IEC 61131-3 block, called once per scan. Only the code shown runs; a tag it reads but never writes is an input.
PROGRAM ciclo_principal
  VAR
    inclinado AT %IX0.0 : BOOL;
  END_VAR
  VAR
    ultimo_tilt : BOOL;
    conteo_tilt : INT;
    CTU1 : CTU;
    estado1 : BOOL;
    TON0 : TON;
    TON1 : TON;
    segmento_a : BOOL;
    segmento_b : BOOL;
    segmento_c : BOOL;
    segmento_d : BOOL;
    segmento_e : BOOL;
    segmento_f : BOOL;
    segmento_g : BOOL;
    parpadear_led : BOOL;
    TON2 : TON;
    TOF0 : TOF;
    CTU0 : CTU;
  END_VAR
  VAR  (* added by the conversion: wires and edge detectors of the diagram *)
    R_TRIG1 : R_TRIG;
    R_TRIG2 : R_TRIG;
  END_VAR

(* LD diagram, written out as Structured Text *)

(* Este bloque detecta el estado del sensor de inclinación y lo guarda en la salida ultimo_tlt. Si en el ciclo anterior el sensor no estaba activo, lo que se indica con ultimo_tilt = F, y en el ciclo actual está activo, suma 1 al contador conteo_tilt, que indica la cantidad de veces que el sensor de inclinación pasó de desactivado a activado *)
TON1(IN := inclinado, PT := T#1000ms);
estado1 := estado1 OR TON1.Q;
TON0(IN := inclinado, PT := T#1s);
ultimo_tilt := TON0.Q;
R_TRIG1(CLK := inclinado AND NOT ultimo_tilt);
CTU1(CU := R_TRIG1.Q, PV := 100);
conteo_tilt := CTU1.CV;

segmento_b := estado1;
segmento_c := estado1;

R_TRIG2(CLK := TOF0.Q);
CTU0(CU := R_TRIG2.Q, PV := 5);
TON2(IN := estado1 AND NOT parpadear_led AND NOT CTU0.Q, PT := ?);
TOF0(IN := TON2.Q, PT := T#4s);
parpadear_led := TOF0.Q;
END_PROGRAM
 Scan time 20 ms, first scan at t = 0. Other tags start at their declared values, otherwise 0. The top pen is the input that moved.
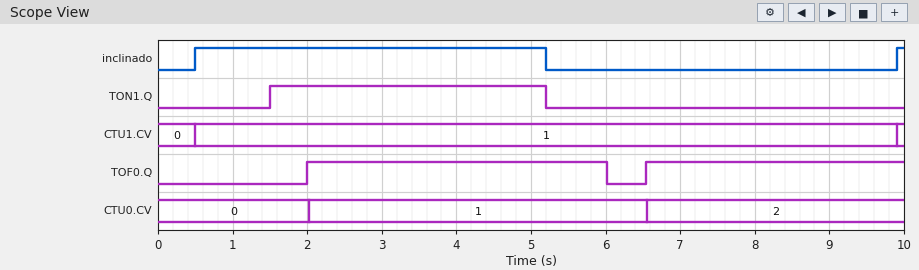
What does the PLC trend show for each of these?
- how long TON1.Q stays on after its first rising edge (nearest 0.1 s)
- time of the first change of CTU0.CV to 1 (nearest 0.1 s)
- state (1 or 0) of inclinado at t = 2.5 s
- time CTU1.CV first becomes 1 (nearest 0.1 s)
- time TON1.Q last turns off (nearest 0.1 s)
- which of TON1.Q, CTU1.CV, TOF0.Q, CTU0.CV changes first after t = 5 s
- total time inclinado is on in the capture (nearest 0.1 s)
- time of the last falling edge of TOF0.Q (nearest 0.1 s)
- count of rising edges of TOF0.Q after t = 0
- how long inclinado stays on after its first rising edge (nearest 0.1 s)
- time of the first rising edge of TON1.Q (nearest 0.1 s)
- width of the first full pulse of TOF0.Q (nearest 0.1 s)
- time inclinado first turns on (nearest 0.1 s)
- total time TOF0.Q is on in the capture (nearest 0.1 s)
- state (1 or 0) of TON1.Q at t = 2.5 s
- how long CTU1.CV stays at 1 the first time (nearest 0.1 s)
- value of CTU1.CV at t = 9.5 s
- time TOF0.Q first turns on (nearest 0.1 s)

3.7 s
2.0 s
1
0.5 s
5.2 s
TON1.Q
4.8 s
6.0 s
2
4.7 s
1.5 s
4.0 s
0.5 s
7.5 s
1
9.4 s
1
2.0 s
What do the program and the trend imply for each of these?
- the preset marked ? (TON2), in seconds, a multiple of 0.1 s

0.5 s
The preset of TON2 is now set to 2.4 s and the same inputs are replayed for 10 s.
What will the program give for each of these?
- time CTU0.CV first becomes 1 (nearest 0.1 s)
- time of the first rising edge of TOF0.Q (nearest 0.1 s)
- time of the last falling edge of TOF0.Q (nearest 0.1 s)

3.9 s
3.9 s
7.9 s
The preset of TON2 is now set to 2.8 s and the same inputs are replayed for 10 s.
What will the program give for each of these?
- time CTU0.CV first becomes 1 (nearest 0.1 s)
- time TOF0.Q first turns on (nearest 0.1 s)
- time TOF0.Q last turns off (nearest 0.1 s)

4.3 s
4.3 s
8.3 s
